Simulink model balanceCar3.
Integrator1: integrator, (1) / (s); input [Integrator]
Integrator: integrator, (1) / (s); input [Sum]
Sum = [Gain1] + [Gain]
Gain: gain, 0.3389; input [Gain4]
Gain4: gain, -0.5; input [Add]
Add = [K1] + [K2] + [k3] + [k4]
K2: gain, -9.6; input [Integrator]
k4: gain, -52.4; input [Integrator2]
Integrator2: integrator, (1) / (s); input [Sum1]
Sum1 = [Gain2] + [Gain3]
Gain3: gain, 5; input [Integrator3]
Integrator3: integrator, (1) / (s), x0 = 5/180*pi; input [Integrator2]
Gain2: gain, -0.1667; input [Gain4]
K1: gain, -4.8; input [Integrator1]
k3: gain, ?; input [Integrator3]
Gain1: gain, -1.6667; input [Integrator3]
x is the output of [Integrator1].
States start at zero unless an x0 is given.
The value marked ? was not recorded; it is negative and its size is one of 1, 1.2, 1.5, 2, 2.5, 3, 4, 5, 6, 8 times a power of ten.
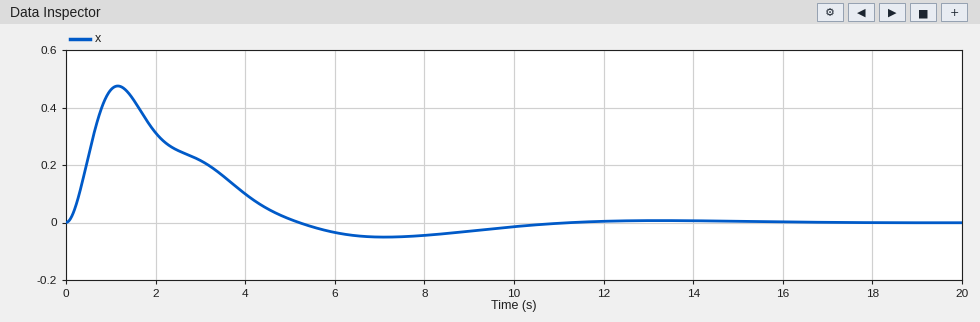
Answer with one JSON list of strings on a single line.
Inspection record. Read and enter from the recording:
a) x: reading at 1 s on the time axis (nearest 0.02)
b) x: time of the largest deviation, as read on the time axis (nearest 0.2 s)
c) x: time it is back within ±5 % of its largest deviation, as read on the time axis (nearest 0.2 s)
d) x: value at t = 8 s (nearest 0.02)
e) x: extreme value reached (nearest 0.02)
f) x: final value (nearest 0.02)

["0.46", "1.2 s", "9.4 s", "-0.04", "0.48", "0.00"]
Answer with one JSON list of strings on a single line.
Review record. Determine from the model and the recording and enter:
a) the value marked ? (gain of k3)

["-200"]
